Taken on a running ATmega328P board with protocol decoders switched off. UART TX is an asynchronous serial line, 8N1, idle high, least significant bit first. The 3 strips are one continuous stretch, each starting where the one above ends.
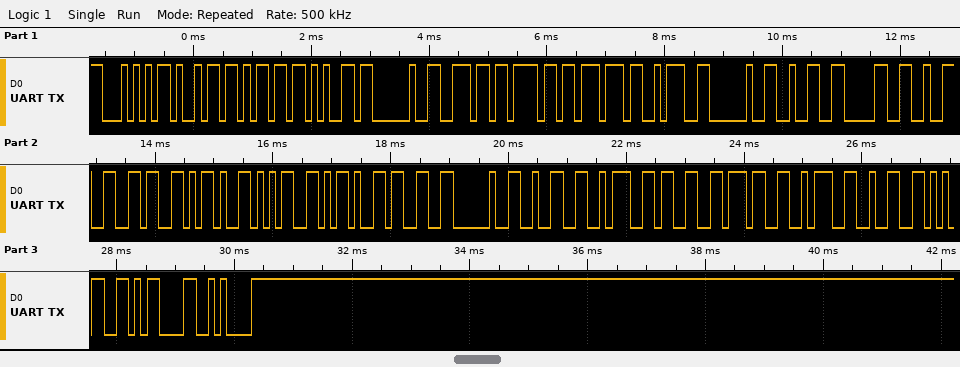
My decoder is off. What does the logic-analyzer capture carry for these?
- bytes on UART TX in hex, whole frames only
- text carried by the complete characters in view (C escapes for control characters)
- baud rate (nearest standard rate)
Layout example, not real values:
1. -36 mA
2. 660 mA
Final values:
1. 54 69 6D 65 20 6E 6F 77 3A 20 32 30 32 36 2D 35 2D 33 20 32 3A 33 37 3A 32 35 0D 0A
2. "Time now: 2026-5-3 2:37:25\r\n"
3. 9600 baud
